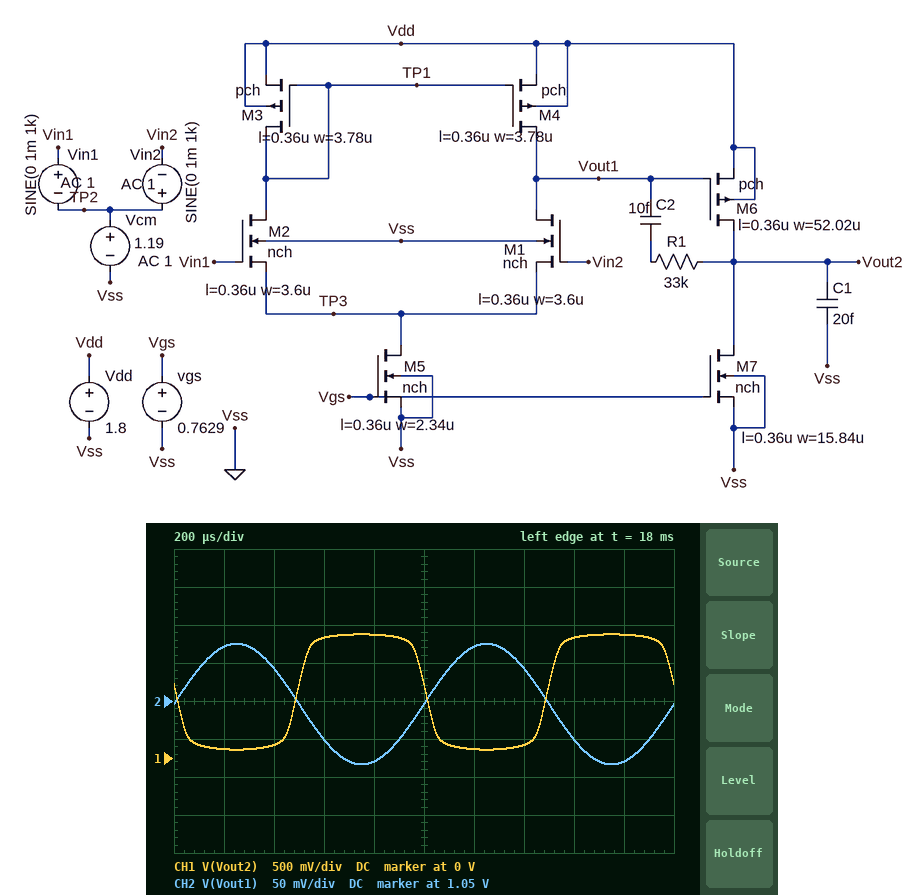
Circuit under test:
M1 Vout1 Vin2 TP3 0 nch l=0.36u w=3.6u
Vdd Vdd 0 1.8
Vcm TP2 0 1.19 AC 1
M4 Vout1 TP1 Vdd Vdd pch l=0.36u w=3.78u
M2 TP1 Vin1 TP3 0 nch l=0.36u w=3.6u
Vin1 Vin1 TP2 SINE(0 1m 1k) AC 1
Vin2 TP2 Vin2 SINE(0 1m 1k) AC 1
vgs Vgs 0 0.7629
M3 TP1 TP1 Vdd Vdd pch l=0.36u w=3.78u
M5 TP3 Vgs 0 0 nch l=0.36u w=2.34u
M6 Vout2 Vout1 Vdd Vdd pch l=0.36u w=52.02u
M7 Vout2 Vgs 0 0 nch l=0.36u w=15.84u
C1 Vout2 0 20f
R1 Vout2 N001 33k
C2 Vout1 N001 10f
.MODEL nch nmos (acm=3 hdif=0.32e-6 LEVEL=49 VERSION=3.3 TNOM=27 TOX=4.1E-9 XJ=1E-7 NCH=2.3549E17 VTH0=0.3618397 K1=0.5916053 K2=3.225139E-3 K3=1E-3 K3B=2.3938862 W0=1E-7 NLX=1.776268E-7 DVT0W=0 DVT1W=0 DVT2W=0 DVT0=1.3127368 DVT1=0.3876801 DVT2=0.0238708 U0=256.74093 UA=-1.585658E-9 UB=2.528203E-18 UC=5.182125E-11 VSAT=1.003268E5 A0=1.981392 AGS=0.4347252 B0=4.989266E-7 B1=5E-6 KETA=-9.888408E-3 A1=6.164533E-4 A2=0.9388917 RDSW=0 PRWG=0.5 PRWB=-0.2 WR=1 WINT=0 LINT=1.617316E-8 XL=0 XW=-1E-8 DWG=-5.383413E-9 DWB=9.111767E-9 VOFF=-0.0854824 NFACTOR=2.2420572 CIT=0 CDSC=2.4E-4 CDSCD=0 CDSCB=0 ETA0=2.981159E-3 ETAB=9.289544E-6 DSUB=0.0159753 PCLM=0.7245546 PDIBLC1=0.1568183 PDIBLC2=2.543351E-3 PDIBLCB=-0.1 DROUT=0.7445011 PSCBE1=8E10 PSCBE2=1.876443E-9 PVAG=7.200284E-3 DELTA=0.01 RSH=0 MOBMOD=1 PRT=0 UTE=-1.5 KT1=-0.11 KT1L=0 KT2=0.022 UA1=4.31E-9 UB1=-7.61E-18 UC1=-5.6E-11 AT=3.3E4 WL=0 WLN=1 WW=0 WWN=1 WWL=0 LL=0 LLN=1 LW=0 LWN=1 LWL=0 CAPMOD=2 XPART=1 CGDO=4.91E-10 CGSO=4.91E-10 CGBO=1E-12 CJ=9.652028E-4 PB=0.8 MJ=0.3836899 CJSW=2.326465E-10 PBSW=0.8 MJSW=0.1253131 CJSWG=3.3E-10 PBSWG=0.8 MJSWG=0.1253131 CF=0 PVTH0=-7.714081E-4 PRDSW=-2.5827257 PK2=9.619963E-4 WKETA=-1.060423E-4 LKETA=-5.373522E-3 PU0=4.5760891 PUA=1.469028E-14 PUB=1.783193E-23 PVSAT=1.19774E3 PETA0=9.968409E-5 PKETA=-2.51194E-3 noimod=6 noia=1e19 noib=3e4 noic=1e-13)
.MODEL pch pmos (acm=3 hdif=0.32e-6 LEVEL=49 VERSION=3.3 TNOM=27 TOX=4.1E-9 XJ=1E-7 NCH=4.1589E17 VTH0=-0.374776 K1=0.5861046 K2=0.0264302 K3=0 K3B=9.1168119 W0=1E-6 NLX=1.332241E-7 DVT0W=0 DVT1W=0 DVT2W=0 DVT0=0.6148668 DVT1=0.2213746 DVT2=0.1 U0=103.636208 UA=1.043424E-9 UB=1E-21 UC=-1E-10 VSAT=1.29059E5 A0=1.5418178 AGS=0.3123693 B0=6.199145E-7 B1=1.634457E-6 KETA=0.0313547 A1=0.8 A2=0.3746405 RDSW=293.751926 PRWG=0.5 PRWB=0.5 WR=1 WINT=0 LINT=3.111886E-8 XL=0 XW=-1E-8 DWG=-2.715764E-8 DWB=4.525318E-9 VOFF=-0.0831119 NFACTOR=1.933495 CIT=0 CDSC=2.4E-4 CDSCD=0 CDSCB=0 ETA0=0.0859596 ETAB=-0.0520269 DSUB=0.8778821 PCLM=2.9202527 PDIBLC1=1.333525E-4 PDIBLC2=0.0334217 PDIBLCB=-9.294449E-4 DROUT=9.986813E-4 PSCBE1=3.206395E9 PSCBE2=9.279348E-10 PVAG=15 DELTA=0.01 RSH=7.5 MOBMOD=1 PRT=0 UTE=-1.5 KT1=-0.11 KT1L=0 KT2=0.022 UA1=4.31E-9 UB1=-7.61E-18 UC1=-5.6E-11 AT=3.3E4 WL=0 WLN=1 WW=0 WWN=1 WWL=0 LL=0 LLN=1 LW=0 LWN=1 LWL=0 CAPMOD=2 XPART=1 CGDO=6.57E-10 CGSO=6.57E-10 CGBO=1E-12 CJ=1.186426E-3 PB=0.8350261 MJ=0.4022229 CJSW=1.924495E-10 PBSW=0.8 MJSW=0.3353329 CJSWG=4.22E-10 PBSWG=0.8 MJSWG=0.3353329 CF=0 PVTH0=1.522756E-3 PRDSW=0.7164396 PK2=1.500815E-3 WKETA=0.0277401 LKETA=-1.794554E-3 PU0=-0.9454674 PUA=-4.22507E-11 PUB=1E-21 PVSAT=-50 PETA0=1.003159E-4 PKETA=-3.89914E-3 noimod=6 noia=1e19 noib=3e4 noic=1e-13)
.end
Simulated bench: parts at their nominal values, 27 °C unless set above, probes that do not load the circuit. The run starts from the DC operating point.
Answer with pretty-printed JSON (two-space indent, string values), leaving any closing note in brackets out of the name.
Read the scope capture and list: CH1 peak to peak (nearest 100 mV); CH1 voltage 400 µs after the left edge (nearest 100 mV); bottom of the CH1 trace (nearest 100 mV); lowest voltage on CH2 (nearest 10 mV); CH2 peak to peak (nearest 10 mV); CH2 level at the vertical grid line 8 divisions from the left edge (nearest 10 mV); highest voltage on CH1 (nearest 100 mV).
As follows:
{
  "CH1 peak to peak": "1.5 V",
  "CH1 voltage 400 µs after the left edge": "200 mV",
  "bottom of the CH1 trace": "100 mV",
  "lowest voltage on CH2": "970 mV",
  "CH2 peak to peak": "160 mV",
  "CH2 level at the vertical grid line 8 divisions from the left edge": "1.00 V",
  "highest voltage on CH1": "1.6 V"
}
